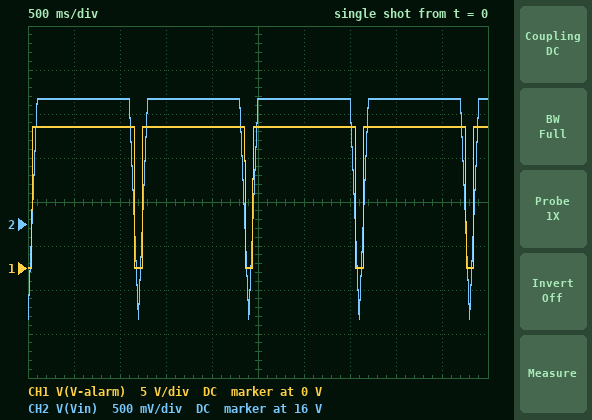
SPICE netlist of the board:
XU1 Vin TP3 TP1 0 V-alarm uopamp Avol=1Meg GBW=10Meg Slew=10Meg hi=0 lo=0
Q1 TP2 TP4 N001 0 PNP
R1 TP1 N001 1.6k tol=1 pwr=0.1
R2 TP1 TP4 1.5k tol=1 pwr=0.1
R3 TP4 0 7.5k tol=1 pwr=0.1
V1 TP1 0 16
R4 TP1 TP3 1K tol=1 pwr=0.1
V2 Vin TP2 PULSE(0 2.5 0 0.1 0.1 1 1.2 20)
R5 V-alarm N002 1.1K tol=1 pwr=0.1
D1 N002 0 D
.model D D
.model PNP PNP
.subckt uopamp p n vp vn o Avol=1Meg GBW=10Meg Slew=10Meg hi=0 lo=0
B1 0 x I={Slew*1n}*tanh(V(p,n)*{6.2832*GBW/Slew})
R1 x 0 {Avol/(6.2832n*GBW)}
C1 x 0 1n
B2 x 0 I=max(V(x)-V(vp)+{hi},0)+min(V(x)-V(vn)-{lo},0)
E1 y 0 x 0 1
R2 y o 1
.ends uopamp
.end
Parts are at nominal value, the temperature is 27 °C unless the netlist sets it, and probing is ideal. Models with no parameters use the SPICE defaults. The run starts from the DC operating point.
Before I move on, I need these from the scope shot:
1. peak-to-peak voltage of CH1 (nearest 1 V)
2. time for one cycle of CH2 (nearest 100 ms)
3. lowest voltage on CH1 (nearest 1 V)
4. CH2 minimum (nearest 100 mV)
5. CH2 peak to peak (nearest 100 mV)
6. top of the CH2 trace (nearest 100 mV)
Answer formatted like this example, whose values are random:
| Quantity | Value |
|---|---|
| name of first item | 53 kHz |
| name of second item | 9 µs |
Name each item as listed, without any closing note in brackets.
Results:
| Quantity | Value |
|---|---|
| peak-to-peak voltage of CH1 | 16 V |
| time for one cycle of CH2 | 1.2 s |
| lowest voltage on CH1 | 0 V |
| CH2 minimum | 14.9 V |
| CH2 peak to peak | 2.5 V |
| top of the CH2 trace | 17.4 V |
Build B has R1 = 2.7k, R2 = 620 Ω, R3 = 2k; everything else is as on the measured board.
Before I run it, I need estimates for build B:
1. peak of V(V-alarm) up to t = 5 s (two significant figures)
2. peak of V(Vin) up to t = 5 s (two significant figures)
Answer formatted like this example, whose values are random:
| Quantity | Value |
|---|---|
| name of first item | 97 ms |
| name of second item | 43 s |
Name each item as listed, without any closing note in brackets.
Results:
| Quantity | Value |
|---|---|
| peak of V(V-alarm) up to t = 5 s | -4.0 mV |
| peak of V(Vin) up to t = 5 s | 16 V |
